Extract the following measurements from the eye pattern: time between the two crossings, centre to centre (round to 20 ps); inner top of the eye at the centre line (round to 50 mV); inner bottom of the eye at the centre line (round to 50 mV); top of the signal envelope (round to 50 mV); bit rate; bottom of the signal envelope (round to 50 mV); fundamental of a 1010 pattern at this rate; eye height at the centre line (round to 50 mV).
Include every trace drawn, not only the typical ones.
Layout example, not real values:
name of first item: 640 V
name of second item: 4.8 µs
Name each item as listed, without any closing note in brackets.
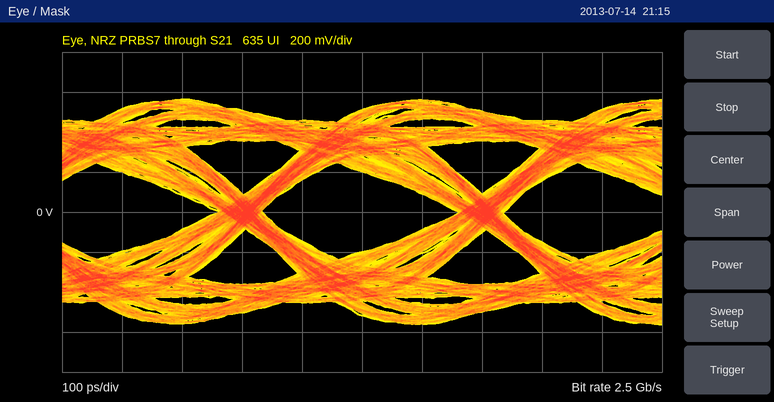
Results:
time between the two crossings, centre to centre: 400 ps
inner top of the eye at the centre line: 200 mV
inner bottom of the eye at the centre line: -200 mV
top of the signal envelope: 550 mV
bit rate: 2.5 Gb/s
bottom of the signal envelope: -550 mV
fundamental of a 1010 pattern at this rate: 1.25 GHz
eye height at the centre line: 400 mV
